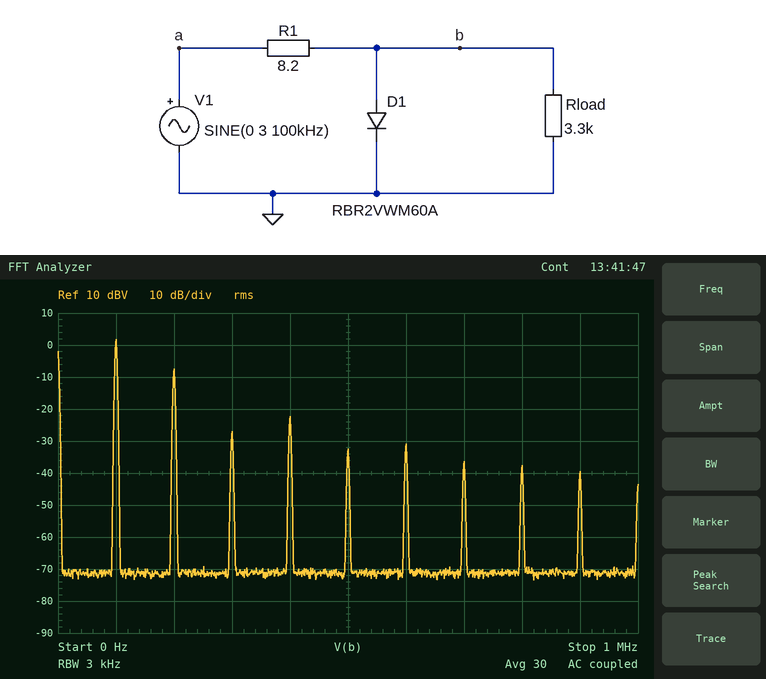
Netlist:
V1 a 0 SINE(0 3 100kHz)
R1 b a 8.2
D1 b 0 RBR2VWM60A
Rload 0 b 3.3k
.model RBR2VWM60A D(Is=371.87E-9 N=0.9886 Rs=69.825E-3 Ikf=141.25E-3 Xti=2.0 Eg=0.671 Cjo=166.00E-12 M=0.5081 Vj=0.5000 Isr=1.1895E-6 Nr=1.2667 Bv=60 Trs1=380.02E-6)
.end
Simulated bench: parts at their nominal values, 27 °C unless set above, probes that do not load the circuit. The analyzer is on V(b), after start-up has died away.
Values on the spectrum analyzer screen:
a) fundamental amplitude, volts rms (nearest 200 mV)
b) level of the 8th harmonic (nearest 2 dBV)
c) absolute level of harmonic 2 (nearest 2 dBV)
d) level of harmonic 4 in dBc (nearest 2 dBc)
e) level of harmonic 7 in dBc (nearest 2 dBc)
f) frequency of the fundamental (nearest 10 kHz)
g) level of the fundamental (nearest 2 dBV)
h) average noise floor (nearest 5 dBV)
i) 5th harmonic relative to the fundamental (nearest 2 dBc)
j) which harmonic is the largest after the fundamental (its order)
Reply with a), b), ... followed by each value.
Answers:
a) 1.2 V
b) -38 dBV
c) -8 dBV
d) -24 dBc
e) -38 dBc
f) 100 kHz
g) 2 dBV
h) -70 dBV
i) -34 dBc
j) 2
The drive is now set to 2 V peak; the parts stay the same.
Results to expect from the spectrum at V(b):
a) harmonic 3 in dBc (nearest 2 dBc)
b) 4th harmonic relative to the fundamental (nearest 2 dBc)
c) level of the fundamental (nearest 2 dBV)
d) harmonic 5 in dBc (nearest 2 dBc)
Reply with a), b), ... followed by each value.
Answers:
a) -26 dBc
b) -26 dBc
c) -2 dBV
d) -32 dBc
